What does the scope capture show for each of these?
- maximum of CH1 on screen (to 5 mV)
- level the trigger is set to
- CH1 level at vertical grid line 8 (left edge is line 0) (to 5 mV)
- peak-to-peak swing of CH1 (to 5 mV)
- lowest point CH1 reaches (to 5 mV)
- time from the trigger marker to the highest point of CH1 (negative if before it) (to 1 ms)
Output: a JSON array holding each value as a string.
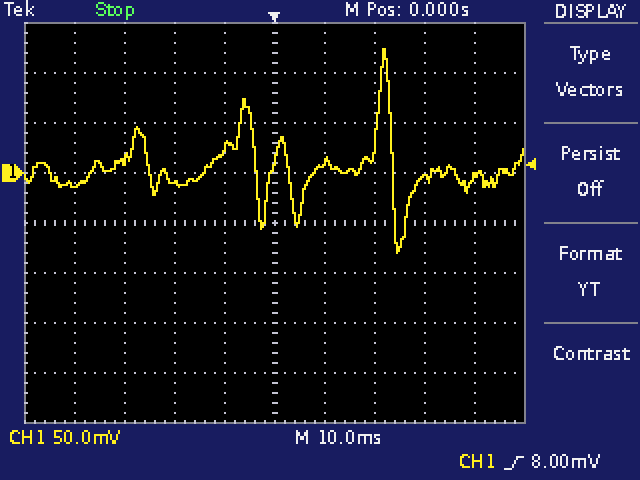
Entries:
["125 mV", "8.00 mV", "-5 mV", "205 mV", "-80 mV", "+22 ms"]
